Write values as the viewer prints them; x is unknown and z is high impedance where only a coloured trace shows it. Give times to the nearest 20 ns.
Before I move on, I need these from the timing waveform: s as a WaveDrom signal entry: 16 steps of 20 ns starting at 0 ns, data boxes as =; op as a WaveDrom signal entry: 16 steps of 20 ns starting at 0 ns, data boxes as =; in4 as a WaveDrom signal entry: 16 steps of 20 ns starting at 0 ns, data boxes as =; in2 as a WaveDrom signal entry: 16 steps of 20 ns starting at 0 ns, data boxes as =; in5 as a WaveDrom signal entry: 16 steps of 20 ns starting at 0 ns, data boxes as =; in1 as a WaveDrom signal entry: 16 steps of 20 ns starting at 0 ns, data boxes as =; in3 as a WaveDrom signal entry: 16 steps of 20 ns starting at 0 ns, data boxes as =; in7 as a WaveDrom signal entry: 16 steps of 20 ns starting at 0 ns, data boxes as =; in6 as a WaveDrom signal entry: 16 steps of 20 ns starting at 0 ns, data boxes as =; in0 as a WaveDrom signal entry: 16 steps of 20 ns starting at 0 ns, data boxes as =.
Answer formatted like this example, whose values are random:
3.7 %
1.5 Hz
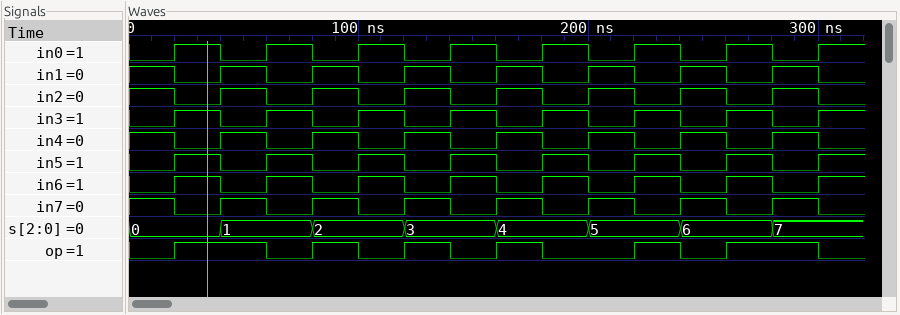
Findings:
{name: 's', wave: '=.=.=.=.=.=.=.=.', data: '0 1 2 3 4 5 6 7'}
{name: 'op', wave: '01.0101010.101.0'}
{name: 'in4', wave: '1010101010101010'}
{name: 'in2', wave: '1010101010101010'}
{name: 'in5', wave: '0101010101010101'}
{name: 'in1', wave: '1010101010101010'}
{name: 'in3', wave: '0101010101010101'}
{name: 'in7', wave: '1010101010101010'}
{name: 'in6', wave: '0101010101010101'}
{name: 'in0', wave: '0101010101010101'}
